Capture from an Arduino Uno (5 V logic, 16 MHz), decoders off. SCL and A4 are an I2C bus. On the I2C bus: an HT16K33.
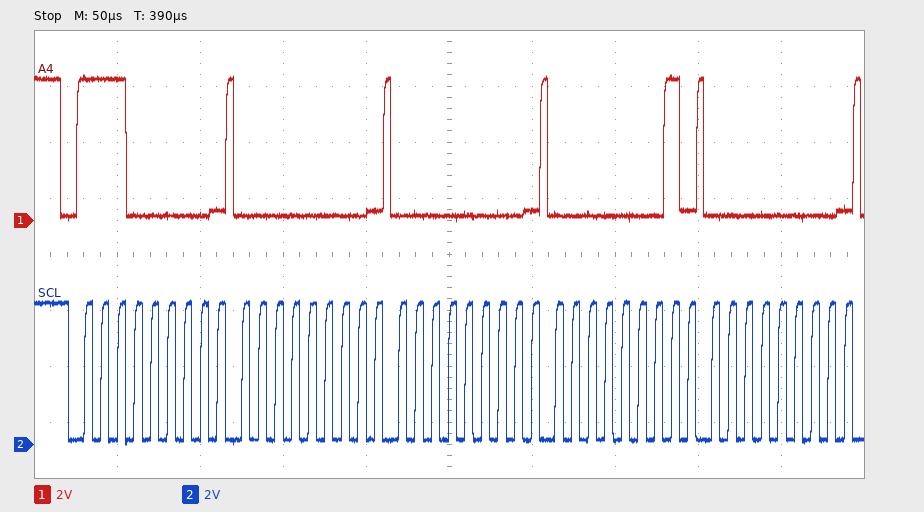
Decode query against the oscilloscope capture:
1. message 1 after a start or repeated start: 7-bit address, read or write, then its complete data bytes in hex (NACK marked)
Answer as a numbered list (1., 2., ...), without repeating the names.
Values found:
1. 0x70 write: 00 00 01 00
